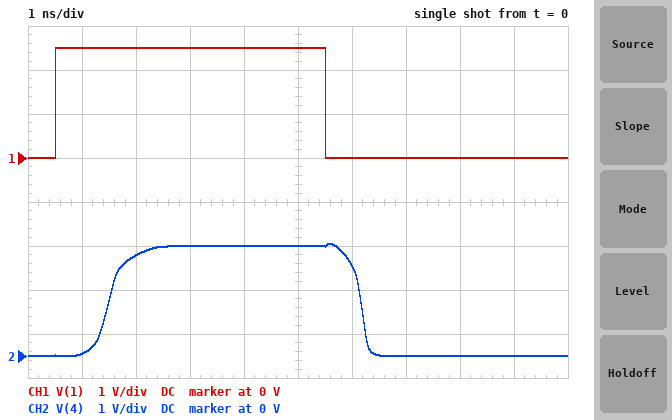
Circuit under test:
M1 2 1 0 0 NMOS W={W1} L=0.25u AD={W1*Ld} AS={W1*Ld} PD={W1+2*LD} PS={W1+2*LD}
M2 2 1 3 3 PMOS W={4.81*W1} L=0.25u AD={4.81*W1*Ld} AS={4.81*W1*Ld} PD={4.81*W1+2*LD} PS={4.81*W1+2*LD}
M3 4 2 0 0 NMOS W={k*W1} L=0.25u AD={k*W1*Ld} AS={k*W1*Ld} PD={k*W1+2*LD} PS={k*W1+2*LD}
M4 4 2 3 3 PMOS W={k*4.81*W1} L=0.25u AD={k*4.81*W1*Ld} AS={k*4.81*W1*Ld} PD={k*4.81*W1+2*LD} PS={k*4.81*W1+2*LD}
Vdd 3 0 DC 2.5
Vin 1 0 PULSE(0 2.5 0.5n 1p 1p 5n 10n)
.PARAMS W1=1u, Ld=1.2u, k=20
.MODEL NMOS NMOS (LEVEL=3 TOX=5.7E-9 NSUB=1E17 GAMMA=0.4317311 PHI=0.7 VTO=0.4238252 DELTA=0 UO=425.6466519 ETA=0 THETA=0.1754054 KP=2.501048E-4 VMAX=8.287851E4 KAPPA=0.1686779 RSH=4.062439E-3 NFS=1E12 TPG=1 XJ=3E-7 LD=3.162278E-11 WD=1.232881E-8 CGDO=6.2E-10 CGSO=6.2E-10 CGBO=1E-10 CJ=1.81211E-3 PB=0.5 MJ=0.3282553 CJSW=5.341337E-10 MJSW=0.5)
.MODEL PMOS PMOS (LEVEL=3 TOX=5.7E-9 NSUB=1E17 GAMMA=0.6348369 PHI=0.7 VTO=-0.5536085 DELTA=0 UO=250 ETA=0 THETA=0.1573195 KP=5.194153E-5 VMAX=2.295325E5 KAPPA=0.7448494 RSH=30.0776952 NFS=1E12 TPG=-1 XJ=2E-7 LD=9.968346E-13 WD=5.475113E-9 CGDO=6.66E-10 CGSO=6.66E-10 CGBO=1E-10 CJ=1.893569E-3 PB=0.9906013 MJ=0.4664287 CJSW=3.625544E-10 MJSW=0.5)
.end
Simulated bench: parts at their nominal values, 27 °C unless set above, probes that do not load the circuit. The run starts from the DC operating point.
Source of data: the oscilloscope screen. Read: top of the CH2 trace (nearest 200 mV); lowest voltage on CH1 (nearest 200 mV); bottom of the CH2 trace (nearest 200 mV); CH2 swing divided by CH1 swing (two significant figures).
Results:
2.6 V
0 V
0 V
1.0
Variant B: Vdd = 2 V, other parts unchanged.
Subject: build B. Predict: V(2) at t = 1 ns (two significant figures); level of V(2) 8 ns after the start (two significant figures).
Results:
1.2 V
2.0 V
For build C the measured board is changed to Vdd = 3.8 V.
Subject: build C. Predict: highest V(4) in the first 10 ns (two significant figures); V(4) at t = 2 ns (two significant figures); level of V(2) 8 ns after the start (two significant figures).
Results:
3.6 V
400 mV
3.8 V
